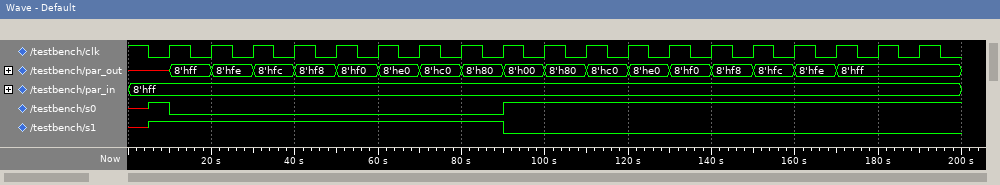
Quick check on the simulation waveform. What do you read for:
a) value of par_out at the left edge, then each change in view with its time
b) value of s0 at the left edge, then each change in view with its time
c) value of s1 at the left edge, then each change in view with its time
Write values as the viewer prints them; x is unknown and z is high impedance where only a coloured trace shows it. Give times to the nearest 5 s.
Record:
x, 8'hff at 10 s, 8'hfe at 20 s, 8'hfc at 30 s, 8'hf8 at 40 s, 8'hf0 at 50 s, 8'he0 at 60 s, 8'hc0 at 70 s, 8'h80 at 80 s, 8'h00 at 90 s, 8'h80 at 100 s, 8'hc0 at 110 s, 8'he0 at 120 s, 8'hf0 at 130 s, 8'hf8 at 140 s, 8'hfc at 150 s, 8'hfe at 160 s, 8'hff at 170 s
x, 1 at 5 s, 0 at 10 s, 1 at 90 s
x, 1 at 5 s, 0 at 90 s
